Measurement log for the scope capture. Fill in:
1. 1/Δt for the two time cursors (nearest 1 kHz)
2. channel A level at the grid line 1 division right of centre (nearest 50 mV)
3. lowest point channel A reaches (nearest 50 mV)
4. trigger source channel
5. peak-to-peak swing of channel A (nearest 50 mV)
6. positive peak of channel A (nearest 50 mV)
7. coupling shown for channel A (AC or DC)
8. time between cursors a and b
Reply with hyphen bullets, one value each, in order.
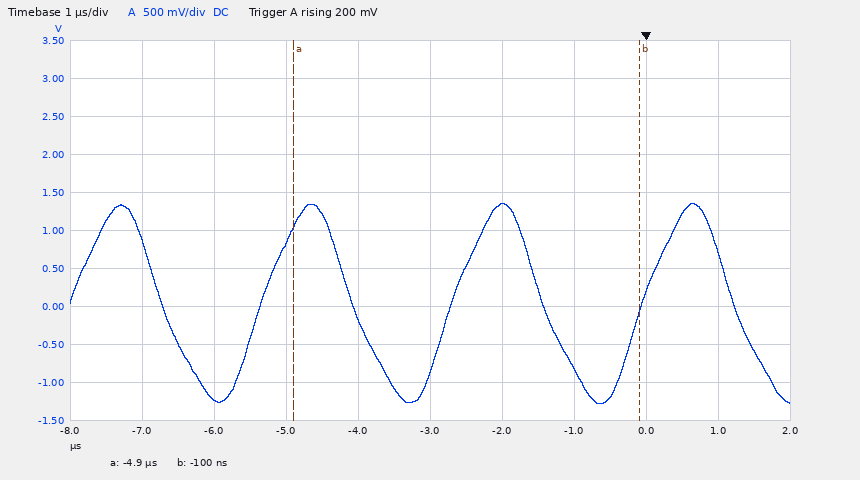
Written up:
- 208 kHz
- 1.35 V
- -1.30 V
- channel A
- 2.65 V
- 1.35 V
- DC
- 4.8 µs
